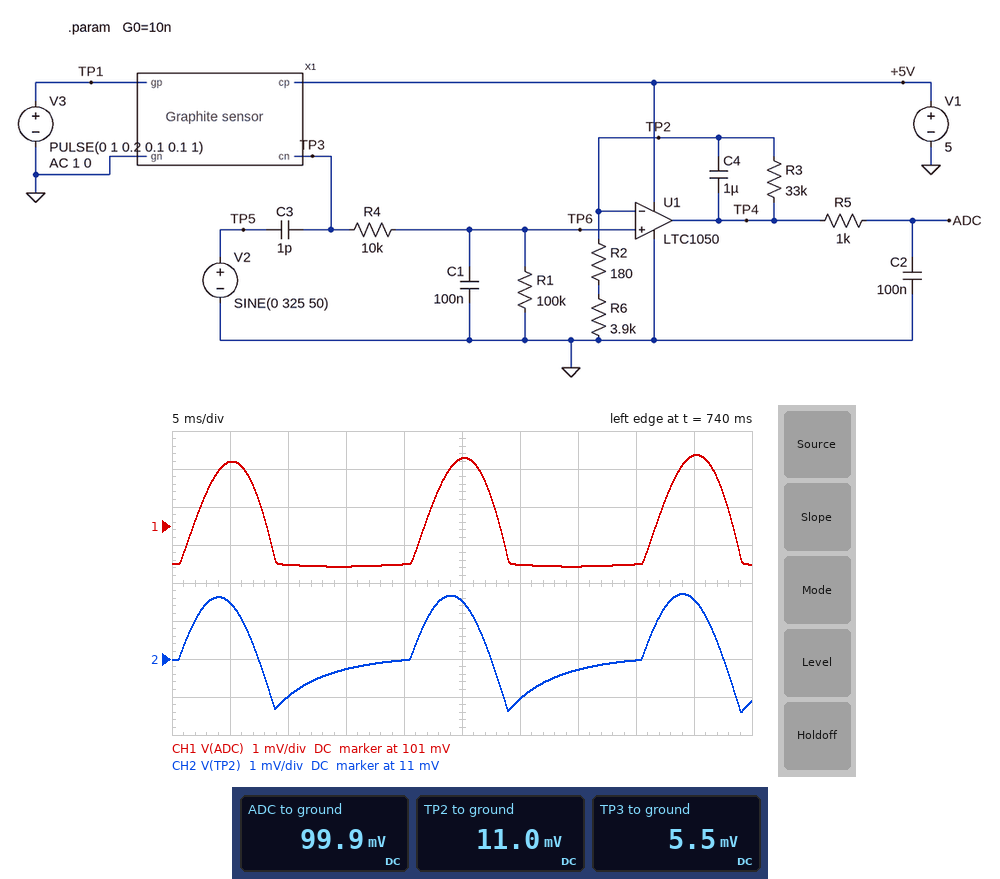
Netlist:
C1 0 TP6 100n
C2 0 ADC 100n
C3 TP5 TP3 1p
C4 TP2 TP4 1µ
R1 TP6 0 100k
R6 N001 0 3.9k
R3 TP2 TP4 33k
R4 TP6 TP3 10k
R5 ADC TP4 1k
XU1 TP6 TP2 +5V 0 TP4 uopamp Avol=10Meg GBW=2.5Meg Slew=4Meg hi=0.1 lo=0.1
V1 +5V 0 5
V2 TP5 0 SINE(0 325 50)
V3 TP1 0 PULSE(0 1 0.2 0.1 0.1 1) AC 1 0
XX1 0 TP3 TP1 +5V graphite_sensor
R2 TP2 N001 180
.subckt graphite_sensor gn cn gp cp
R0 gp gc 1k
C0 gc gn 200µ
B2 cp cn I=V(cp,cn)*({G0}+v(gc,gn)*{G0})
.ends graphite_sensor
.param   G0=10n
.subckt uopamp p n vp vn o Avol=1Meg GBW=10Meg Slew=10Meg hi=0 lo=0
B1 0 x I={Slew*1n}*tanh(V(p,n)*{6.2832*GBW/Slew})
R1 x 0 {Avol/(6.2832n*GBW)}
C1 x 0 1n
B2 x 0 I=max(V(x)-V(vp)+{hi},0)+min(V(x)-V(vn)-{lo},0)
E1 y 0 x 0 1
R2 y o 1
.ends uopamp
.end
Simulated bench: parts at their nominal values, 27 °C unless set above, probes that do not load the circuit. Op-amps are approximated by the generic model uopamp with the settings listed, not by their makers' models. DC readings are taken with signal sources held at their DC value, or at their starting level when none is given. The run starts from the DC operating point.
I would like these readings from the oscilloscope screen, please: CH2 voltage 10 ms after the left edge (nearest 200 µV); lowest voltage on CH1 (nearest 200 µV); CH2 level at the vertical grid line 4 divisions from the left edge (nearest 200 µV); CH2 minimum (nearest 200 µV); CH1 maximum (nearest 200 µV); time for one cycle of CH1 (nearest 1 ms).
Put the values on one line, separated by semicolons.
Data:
10.0 mV; 100.0 mV; 11.0 mV; 9.6 mV; 102.8 mV; 20 ms
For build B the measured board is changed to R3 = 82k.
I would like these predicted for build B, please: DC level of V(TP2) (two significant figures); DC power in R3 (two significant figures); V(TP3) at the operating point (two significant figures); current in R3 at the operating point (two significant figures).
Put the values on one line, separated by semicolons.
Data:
5.0 mV; 120 nW; 5.5 mV; 1.2 µA
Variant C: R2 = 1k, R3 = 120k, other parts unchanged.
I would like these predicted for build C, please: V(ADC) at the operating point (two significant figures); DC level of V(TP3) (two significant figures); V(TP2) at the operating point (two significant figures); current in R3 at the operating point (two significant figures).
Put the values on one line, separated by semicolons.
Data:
130 mV; 5.5 mV; 5.0 mV; 1.0 µA
